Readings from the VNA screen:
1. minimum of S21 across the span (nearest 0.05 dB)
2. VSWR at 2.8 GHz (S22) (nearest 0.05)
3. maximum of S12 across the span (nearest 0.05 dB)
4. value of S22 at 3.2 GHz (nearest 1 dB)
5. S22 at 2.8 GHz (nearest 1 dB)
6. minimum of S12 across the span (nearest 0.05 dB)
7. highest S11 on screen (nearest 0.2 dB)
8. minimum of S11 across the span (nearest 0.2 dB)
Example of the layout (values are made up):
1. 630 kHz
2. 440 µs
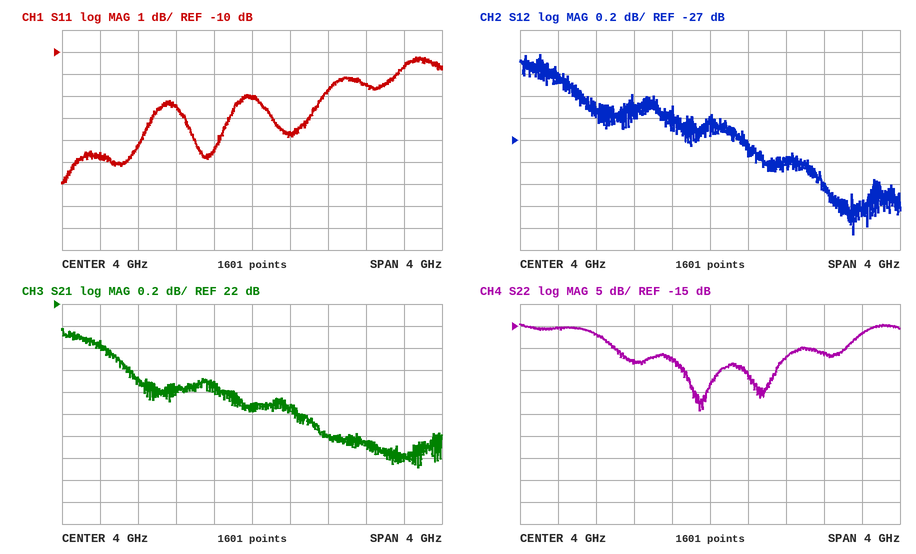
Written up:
1. 20.50 dB
2. 1.35
3. -26.20 dB
4. -23 dB
5. -17 dB
6. -27.85 dB
7. -10.2 dB
8. -16.0 dB
